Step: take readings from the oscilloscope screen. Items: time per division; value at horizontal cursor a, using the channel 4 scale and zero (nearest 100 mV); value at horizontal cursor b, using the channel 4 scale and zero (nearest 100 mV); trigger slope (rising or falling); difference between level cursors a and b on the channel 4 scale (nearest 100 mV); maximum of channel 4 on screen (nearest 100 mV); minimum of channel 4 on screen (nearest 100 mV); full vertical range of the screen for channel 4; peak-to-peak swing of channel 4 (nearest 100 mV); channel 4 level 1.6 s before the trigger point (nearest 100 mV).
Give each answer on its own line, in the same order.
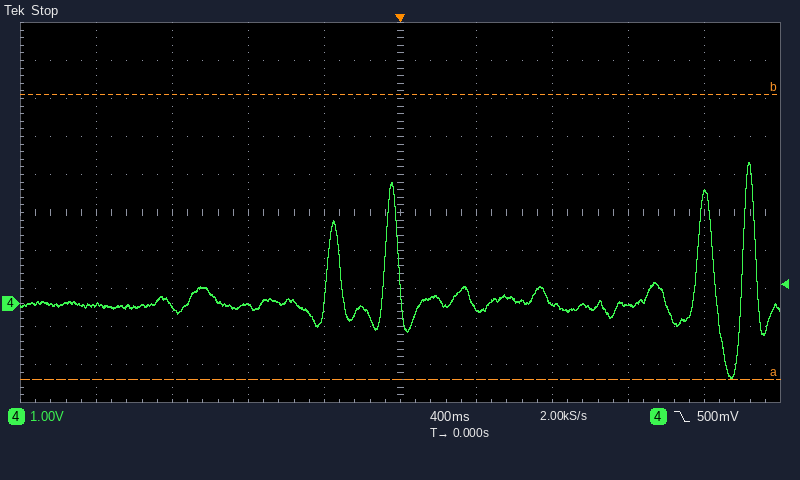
400 ms
-2.0 V
5.5 V
falling
7.5 V
3.7 V
-2.0 V
10 V
5.7 V
0.0 V
